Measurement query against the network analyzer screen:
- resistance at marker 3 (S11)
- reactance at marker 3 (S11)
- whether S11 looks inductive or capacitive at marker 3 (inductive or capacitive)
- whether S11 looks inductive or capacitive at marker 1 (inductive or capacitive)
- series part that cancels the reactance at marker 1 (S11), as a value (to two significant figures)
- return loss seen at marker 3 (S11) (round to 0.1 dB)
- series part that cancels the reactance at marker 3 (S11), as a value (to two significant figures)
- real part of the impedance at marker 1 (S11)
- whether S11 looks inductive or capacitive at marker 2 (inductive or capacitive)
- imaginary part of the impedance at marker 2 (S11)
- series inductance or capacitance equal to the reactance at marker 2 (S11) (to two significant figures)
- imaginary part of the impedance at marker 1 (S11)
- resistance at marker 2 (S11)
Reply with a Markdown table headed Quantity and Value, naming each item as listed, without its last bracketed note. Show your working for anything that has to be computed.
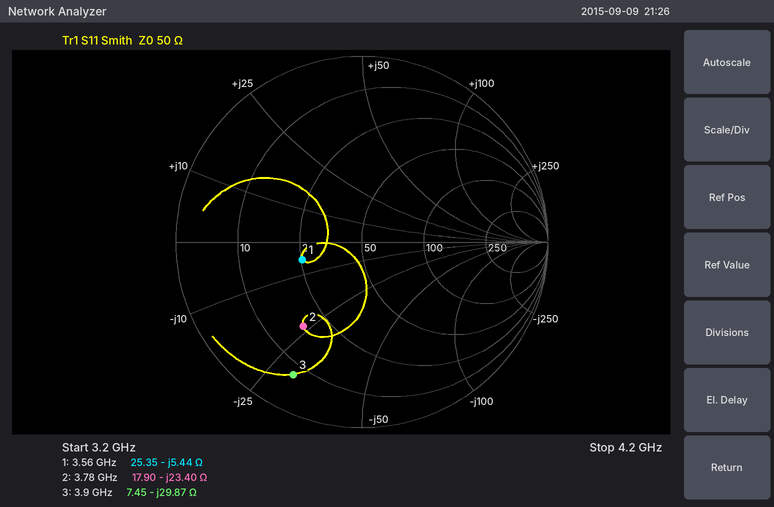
| Quantity | Value |
|---|---|
| resistance at marker 3 | 7.45 Ω |
| reactance at marker 3 | -29.87 Ω |
| whether S11 looks inductive or capacitive at marker 3 | capacitive |
| whether S11 looks inductive or capacitive at marker 1 | capacitive |
| series part that cancels the reactance at marker 1 (S11), as a value | L = 5.44 Ω/(2π × 3.56 GHz) ≈ 243 pH, so 240 pH to two significant figures |
| return loss seen at marker 3 (S11) | 1.9 dB |
| series part that cancels the reactance at marker 3 (S11), as a value | L = 29.87 Ω/(2π × 3.9 GHz) ≈ 1.2 nH |
| real part of the impedance at marker 1 | 25.35 Ω |
| whether S11 looks inductive or capacitive at marker 2 | capacitive |
| imaginary part of the impedance at marker 2 | -23.40 Ω |
| series inductance or capacitance equal to the reactance at marker 2 (S11) | C = 1/(2π × 3.78 GHz × 23.4 Ω) ≈ 1.8 pF |
| imaginary part of the impedance at marker 1 | -5.44 Ω |
| resistance at marker 2 | 17.90 Ω |
